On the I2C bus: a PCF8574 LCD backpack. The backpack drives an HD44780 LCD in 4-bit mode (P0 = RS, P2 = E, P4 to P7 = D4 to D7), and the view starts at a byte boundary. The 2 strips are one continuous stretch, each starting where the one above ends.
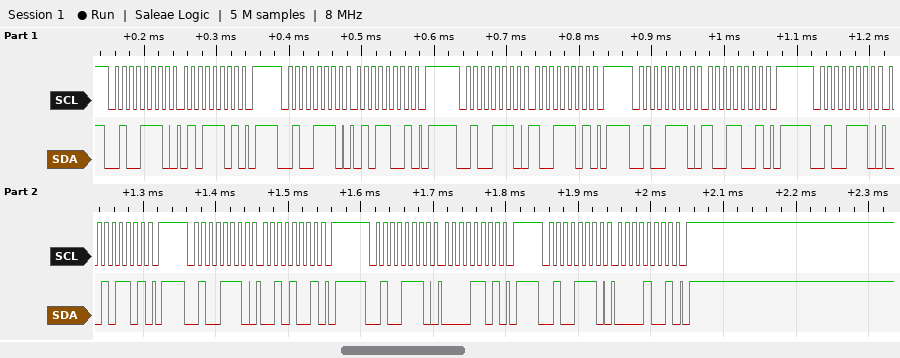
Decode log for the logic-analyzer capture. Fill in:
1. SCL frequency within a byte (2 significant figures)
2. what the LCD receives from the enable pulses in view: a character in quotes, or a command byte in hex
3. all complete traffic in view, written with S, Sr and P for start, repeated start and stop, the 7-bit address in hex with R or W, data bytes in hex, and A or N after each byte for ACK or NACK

100 kHz
'Y' ' '
S 27W A 5D A P S 27W A 59 A P S 27W A 9D A P S 27W A 99 A P S 27W A 2D A P S 27W A 29 A P S 27W A 0D A P S 27W A 09 A P
